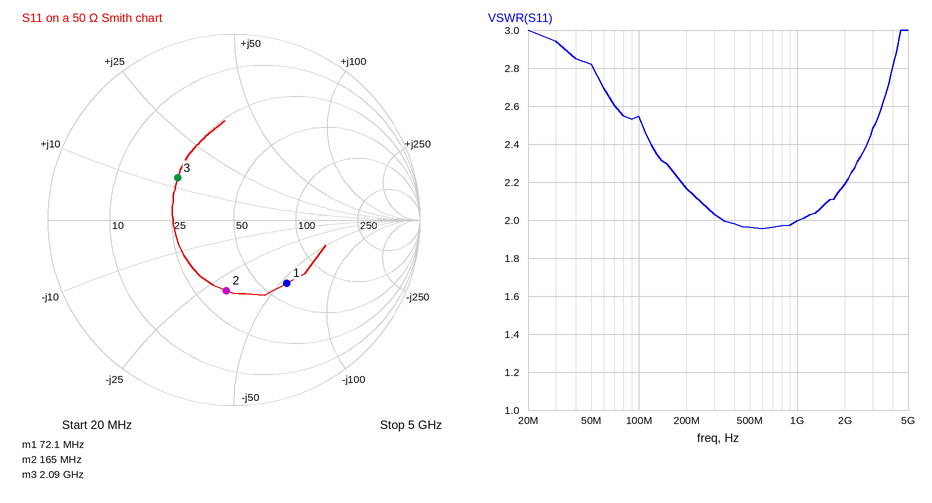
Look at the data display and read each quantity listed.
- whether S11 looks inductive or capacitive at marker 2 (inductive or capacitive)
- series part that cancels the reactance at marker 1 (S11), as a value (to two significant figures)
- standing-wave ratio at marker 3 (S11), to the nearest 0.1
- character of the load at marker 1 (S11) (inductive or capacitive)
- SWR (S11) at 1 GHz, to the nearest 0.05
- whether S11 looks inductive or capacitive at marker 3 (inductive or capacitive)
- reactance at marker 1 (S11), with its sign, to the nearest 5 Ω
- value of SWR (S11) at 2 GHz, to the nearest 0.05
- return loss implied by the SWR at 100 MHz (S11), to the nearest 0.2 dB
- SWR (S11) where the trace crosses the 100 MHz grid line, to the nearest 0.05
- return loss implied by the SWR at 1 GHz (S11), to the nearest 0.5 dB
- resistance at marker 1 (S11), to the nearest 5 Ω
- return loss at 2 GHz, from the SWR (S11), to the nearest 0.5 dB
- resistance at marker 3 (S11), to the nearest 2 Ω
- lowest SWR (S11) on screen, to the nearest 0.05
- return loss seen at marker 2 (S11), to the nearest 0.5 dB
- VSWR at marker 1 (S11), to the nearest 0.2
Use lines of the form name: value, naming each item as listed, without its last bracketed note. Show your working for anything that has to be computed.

whether S11 looks inductive or capacitive at marker 2: capacitive
series part that cancels the reactance at marker 1 (S11), as a value: L = 55 Ω/(2π × 72.1 MHz) ≈ 121 nH, so 120 nH to two significant figures
standing-wave ratio at marker 3 (S11), to the nearest 0.1: 2.2
character of the load at marker 1 (S11): capacitive
SWR (S11) at 1 GHz, to the nearest 0.05: 2.00
whether S11 looks inductive or capacitive at marker 3: inductive
reactance at marker 1 (S11), with its sign, to the nearest 5 Ω: -55 Ω
value of SWR (S11) at 2 GHz, to the nearest 0.05: 2.20
return loss implied by the SWR at 100 MHz (S11), to the nearest 0.2 dB: −20 log10((2.55 − 1)/(2.55 + 1)) ≈ 7.2 dB
SWR (S11) where the trace crosses the 100 MHz grid line, to the nearest 0.05: 2.55
return loss implied by the SWR at 1 GHz (S11), to the nearest 0.5 dB: −20 log10((2 − 1)/(2 + 1)) ≈ 9.5 dB
resistance at marker 1 (S11), to the nearest 5 Ω: 65 Ω
return loss at 2 GHz, from the SWR (S11), to the nearest 0.5 dB: −20 log10((2.2 − 1)/(2.2 + 1)) ≈ 8.5 dB
resistance at marker 3 (S11), to the nearest 2 Ω: 24 Ω
lowest SWR (S11) on screen, to the nearest 0.05: 1.95
return loss seen at marker 2 (S11), to the nearest 0.5 dB: 8.5 dB
VSWR at marker 1 (S11), to the nearest 0.2: 2.6
